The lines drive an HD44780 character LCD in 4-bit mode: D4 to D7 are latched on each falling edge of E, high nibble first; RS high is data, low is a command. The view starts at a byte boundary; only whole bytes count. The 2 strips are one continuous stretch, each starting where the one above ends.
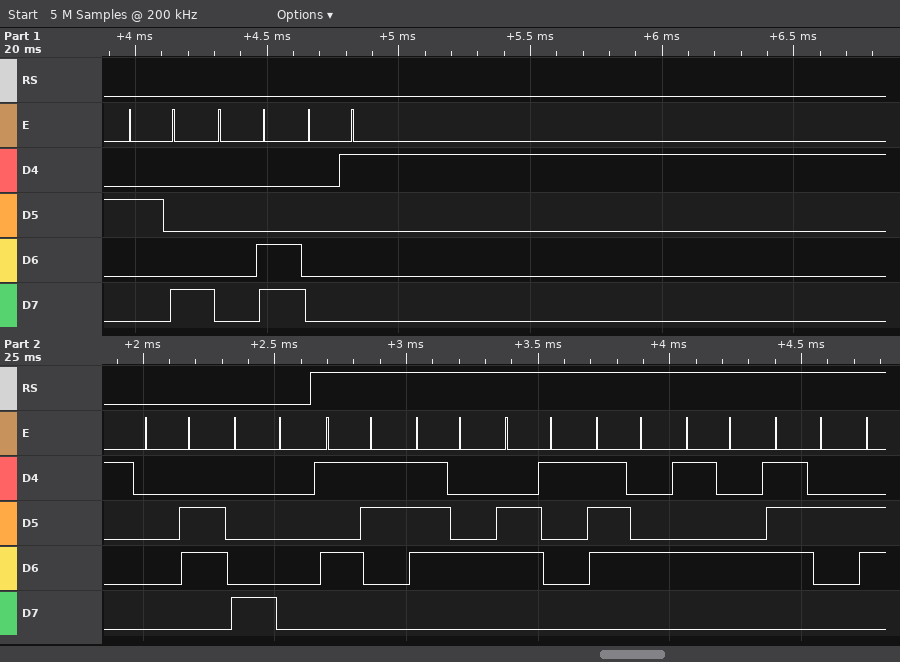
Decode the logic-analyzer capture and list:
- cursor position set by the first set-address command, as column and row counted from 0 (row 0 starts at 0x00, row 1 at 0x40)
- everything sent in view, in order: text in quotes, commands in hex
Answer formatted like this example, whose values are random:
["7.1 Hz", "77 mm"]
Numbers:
["column 0, row 0", "0x28 0x0C 0x01 0x06 0x80 \"StatTr\""]
